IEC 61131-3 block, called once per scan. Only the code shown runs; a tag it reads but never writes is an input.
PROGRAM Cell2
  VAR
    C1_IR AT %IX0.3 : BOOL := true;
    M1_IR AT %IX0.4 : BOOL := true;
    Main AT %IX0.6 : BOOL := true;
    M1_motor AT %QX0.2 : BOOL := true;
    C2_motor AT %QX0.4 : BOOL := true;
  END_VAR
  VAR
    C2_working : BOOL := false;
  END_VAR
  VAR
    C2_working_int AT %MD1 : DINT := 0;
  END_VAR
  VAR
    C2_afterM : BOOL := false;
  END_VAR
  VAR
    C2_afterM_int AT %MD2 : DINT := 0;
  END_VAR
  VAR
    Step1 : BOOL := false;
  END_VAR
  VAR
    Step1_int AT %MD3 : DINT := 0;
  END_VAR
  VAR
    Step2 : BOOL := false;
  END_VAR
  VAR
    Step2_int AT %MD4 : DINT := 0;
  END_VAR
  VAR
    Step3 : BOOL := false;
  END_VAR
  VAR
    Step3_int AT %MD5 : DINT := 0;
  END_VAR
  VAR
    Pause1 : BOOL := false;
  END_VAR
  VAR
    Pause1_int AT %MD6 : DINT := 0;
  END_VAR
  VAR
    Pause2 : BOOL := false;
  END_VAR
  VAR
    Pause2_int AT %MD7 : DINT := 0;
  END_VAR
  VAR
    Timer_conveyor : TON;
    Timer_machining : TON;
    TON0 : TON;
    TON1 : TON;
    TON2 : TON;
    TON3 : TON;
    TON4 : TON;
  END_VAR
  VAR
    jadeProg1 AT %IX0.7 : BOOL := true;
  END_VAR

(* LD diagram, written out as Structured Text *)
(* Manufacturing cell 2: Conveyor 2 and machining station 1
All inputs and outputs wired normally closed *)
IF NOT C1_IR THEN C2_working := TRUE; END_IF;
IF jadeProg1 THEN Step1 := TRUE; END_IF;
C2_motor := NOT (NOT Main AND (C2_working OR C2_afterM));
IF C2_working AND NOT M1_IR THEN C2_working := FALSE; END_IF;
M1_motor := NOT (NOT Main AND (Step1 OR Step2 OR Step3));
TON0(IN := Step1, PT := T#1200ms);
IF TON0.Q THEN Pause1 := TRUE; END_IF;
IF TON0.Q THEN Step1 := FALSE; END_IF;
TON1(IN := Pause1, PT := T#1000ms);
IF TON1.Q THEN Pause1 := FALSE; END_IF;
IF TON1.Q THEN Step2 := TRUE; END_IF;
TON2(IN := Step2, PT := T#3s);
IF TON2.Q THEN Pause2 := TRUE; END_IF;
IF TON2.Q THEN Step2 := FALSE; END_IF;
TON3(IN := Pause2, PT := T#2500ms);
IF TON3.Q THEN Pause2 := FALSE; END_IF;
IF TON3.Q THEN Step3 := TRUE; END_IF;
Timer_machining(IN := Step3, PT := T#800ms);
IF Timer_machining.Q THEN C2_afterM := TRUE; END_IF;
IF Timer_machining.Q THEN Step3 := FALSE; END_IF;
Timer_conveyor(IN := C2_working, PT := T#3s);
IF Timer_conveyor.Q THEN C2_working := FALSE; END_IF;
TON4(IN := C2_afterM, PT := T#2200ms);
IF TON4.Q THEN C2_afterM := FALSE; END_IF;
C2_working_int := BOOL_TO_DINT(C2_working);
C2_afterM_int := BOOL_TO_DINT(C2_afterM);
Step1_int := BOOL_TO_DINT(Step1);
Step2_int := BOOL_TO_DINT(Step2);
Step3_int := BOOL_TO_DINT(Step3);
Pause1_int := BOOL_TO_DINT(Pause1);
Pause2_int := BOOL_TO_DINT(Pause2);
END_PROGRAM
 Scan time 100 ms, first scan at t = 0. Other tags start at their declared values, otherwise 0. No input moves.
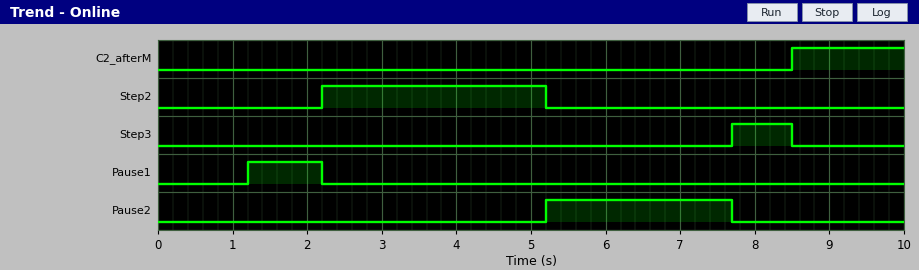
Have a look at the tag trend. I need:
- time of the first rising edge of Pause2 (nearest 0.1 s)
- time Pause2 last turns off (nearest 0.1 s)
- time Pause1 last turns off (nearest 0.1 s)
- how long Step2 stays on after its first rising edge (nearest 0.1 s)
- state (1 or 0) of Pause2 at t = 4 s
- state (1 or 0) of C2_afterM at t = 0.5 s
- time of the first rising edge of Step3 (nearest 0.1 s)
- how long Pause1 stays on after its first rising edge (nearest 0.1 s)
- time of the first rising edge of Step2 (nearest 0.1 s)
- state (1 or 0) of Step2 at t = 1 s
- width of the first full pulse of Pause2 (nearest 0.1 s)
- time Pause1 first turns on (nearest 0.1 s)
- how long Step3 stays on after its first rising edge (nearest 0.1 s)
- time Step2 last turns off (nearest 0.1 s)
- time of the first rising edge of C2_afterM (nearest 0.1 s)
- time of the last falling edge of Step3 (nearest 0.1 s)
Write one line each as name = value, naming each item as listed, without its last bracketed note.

time of the first rising edge of Pause2 = 5.2 s
time Pause2 last turns off = 7.7 s
time Pause1 last turns off = 2.2 s
how long Step2 stays on after its first rising edge = 3.0 s
state (1 or 0) of Pause2 at t = 4 s = 0
state (1 or 0) of C2_afterM at t = 0.5 s = 0
time of the first rising edge of Step3 = 7.7 s
how long Pause1 stays on after its first rising edge = 1.0 s
time of the first rising edge of Step2 = 2.2 s
state (1 or 0) of Step2 at t = 1 s = 0
width of the first full pulse of Pause2 = 2.5 s
time Pause1 first turns on = 1.2 s
how long Step3 stays on after its first rising edge = 0.8 s
time Step2 last turns off = 5.2 s
time of the first rising edge of C2_afterM = 8.5 s
time of the last falling edge of Step3 = 8.5 s
